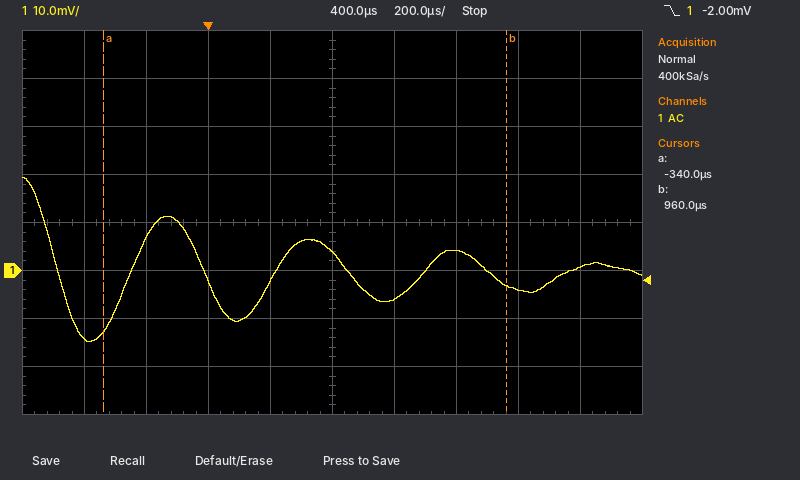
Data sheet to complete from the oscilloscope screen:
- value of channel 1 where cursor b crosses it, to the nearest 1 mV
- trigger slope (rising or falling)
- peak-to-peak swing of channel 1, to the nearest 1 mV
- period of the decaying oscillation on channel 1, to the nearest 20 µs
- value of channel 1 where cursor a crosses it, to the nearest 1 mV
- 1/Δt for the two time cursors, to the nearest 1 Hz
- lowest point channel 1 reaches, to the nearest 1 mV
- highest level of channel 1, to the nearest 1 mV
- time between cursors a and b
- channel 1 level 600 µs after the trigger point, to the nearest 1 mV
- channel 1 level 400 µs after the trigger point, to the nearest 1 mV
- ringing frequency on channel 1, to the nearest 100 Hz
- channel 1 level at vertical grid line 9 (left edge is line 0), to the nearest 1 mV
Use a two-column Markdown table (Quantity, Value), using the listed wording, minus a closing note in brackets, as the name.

| Quantity | Value |
|---|---|
| value of channel 1 where cursor b crosses it, to the nearest 1 mV | -3 mV |
| trigger slope | falling |
| peak-to-peak swing of channel 1, to the nearest 1 mV | 34 mV |
| period of the decaying oscillation on channel 1, to the nearest 20 µs | 460 µs |
| value of channel 1 where cursor a crosses it, to the nearest 1 mV | -13 mV |
| 1/Δt for the two time cursors, to the nearest 1 Hz | 769 Hz |
| lowest point channel 1 reaches, to the nearest 1 mV | -15 mV |
| highest level of channel 1, to the nearest 1 mV | 19 mV |
| time between cursors a and b | 1.30 ms |
| channel 1 level 600 µs after the trigger point, to the nearest 1 mV | -6 mV |
| channel 1 level 400 µs after the trigger point, to the nearest 1 mV | 4 mV |
| ringing frequency on channel 1, to the nearest 100 Hz | 2.2 kHz |
| channel 1 level at vertical grid line 9 (left edge is line 0), to the nearest 1 mV | 1 mV |
